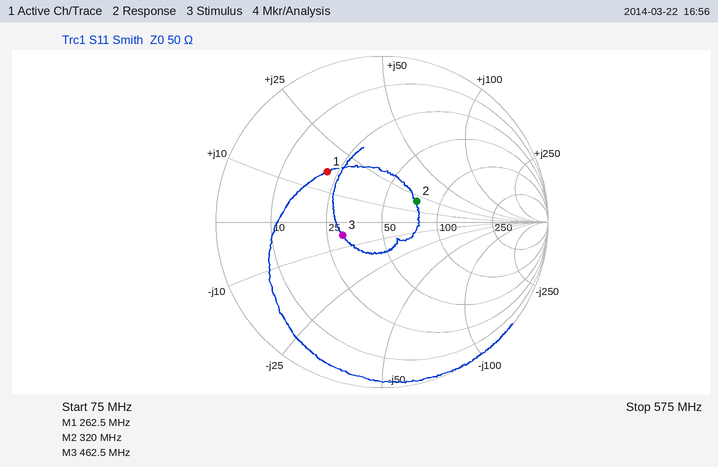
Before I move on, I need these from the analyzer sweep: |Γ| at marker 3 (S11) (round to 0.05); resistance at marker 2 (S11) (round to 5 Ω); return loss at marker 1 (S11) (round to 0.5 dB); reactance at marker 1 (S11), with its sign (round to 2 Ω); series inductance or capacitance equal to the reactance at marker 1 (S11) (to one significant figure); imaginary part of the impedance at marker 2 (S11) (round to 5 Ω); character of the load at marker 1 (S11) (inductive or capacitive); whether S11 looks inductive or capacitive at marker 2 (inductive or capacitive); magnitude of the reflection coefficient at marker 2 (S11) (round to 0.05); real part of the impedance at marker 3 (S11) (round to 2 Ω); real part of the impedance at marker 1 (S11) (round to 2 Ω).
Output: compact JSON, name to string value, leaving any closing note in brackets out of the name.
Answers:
{"|Γ| at marker 3 (S11)": "0.25", "resistance at marker 2 (S11)": "75 Ω", "return loss at marker 1 (S11)": "7.0 dB", "reactance at marker 1 (S11), with its sign": "+16 Ω", "series inductance or capacitance equal to the reactance at marker 1 (S11)": "10 nH", "imaginary part of the impedance at marker 2 (S11)": "+20 Ω", "character of the load at marker 1 (S11)": "inductive", "whether S11 looks inductive or capacitive at marker 2": "inductive", "magnitude of the reflection coefficient at marker 2 (S11)": "0.25", "real part of the impedance at marker 3 (S11)": "30 Ω", "real part of the impedance at marker 1 (S11)": "22 Ω"}
